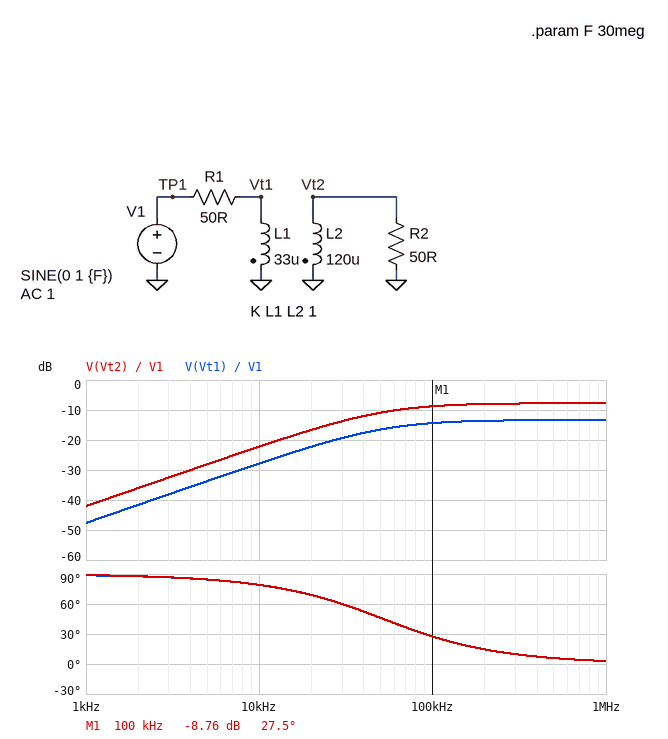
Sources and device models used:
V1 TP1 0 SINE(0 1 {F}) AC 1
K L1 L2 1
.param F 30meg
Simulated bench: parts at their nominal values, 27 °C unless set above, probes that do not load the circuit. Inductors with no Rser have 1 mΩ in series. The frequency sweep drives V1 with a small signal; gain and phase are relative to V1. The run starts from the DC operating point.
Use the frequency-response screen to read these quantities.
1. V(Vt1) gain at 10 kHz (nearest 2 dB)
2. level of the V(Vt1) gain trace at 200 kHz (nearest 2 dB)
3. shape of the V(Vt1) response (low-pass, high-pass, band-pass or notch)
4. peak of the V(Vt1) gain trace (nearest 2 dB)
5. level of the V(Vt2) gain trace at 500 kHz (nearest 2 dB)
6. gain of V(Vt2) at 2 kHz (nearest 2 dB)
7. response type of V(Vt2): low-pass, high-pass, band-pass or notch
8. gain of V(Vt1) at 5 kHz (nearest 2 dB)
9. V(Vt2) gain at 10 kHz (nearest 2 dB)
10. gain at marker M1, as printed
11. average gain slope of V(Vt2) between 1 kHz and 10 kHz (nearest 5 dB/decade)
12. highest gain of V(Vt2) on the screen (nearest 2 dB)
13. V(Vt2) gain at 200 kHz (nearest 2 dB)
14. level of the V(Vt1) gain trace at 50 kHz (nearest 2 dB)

-28 dB
-14 dB
high-pass
-14 dB
-8 dB
-36 dB
high-pass
-34 dB
-22 dB
-8.76 dB
20 dB/decade
-8 dB
-8 dB
-16 dB
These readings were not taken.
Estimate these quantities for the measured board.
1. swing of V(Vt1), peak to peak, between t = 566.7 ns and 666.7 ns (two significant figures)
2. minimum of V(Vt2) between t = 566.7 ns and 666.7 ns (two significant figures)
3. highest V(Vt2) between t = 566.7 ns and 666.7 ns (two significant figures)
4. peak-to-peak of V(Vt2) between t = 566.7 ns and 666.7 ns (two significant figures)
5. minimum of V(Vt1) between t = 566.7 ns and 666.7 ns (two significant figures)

430 mV
-410 mV
410 mV
820 mV
-220 mV
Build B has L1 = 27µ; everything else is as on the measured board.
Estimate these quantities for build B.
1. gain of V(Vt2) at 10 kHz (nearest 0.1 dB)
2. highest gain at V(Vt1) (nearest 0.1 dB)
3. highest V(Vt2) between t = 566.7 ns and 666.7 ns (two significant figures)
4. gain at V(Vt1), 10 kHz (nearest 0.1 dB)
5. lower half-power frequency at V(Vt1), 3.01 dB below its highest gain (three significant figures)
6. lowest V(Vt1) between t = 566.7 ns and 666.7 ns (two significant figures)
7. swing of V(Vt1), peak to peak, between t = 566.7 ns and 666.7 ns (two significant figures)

-23.1 dB
-14.7 dB
390 mV
-29.5 dB
54.1 kHz
-180 mV
370 mV
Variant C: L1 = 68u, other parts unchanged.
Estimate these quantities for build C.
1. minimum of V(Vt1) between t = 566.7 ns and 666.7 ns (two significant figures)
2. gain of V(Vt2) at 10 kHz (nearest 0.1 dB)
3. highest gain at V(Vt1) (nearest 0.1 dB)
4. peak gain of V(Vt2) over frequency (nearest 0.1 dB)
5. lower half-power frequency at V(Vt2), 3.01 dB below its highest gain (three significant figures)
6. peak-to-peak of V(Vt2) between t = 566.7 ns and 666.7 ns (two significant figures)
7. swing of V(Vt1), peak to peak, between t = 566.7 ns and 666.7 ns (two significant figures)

-360 mV
-19.1 dB
-8.8 dB
-6.4 dB
42.3 kHz
960 mV
720 mV
